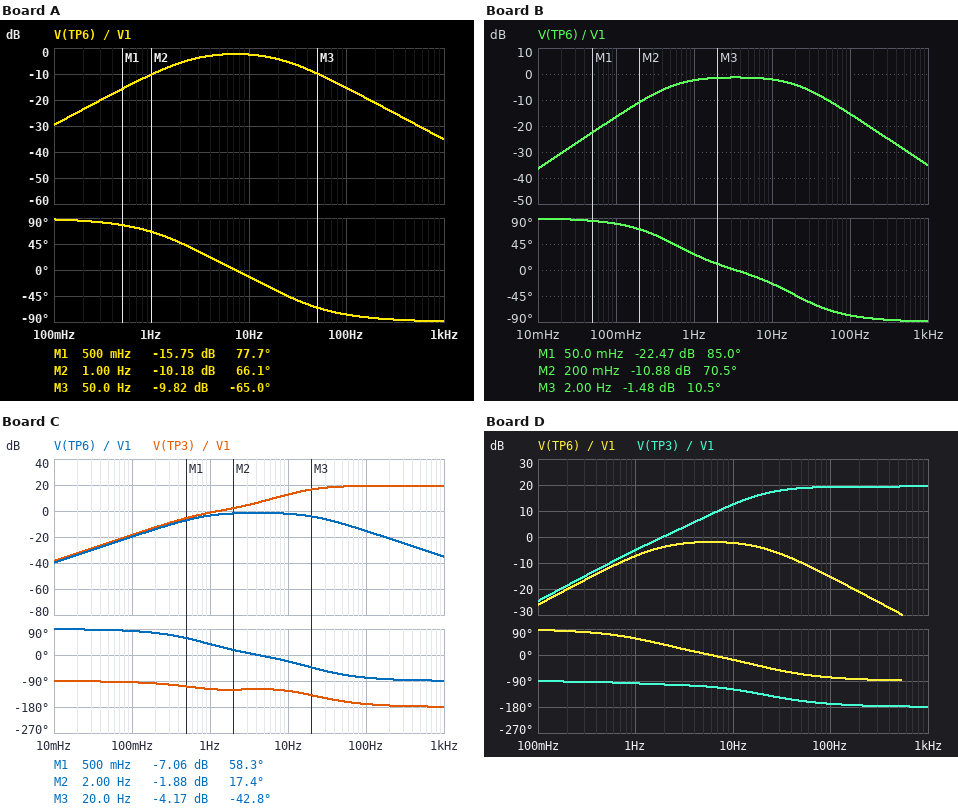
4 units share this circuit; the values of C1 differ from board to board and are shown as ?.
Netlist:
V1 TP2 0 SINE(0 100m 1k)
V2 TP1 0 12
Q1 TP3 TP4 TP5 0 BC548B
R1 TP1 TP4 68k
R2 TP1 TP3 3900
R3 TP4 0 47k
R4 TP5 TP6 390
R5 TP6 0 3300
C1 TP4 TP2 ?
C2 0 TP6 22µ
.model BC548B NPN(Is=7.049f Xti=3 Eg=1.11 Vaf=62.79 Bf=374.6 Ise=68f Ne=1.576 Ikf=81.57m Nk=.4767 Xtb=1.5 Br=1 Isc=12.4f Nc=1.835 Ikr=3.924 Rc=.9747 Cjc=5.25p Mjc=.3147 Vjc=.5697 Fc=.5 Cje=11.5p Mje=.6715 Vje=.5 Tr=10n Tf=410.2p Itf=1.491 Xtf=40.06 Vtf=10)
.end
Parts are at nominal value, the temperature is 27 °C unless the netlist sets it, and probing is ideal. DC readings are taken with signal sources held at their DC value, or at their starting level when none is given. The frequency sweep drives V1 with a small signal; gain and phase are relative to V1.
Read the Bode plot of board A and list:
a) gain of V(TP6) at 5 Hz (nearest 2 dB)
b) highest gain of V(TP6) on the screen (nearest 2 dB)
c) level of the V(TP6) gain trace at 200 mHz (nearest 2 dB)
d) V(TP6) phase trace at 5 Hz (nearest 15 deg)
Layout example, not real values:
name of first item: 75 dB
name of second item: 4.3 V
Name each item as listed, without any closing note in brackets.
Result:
gain of V(TP6) at 5 Hz: -2 dB
highest gain of V(TP6) on the screen: -2 dB
level of the V(TP6) gain trace at 200 mHz: -24 dB
V(TP6) phase trace at 5 Hz: 15 deg
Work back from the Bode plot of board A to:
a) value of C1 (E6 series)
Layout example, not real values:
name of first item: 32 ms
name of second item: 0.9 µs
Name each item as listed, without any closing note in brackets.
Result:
value of C1: 2.2 µF
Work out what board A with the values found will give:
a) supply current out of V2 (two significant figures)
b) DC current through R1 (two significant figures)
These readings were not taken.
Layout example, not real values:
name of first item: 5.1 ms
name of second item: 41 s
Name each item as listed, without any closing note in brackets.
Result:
supply current out of V2: 1.2 mA
DC current through R1: 110 µA
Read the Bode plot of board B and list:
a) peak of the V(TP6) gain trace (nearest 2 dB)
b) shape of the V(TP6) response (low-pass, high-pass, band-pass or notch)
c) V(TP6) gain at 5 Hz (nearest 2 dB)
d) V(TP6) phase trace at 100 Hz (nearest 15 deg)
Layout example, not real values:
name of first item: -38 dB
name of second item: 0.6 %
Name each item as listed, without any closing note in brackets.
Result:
peak of the V(TP6) gain trace: -2 dB
shape of the V(TP6) response: band-pass
V(TP6) gain at 5 Hz: -2 dB
V(TP6) phase trace at 100 Hz: -75 deg
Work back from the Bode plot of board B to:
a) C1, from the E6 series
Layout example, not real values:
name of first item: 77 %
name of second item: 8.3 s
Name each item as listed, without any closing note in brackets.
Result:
C1, from the E6 series: 10 µF
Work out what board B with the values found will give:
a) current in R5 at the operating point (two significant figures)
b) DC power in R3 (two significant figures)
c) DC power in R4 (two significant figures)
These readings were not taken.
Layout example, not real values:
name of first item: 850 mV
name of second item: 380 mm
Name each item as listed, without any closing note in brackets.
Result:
current in R5 at the operating point: 1.1 mA
DC power in R3: 490 µW
DC power in R4: 490 µW
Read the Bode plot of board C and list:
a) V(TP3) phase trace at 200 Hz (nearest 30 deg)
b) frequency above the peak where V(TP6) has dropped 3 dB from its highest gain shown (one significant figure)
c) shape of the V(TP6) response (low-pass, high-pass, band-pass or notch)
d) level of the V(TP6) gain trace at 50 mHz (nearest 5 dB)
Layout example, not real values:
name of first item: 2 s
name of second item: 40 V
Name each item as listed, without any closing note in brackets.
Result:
V(TP3) phase trace at 200 Hz: -180 deg
frequency above the peak where V(TP6) has dropped 3 dB from its highest gain shown: 20 Hz
shape of the V(TP6) response: band-pass
level of the V(TP6) gain trace at 50 mHz: -25 dB
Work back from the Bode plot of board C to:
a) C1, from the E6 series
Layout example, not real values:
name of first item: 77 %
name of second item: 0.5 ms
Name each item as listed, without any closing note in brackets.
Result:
C1, from the E6 series: 6.8 µF
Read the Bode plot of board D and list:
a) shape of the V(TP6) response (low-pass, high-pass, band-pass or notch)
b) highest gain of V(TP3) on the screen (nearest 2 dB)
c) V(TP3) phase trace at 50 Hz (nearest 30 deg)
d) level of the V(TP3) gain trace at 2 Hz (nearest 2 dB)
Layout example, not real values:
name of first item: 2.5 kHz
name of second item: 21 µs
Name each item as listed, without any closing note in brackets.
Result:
shape of the V(TP6) response: band-pass
highest gain of V(TP3) on the screen: 20 dB
V(TP3) phase trace at 50 Hz: -150 deg
level of the V(TP3) gain trace at 2 Hz: 0 dB
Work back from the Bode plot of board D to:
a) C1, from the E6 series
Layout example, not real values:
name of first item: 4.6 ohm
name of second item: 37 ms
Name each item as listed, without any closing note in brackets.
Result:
C1, from the E6 series: 3.3 µF
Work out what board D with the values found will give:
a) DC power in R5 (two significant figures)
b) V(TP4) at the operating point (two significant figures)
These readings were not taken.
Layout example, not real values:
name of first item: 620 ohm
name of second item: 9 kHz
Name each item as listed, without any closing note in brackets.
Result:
DC power in R5: 4.1 mW
V(TP4) at the operating point: 4.8 V
